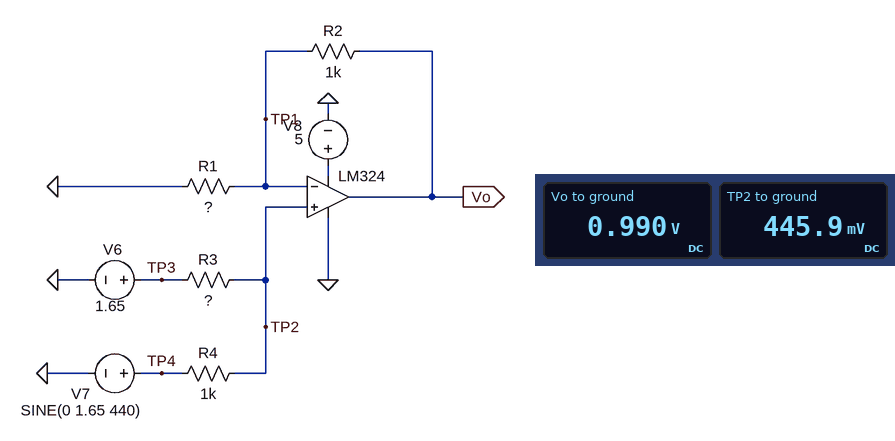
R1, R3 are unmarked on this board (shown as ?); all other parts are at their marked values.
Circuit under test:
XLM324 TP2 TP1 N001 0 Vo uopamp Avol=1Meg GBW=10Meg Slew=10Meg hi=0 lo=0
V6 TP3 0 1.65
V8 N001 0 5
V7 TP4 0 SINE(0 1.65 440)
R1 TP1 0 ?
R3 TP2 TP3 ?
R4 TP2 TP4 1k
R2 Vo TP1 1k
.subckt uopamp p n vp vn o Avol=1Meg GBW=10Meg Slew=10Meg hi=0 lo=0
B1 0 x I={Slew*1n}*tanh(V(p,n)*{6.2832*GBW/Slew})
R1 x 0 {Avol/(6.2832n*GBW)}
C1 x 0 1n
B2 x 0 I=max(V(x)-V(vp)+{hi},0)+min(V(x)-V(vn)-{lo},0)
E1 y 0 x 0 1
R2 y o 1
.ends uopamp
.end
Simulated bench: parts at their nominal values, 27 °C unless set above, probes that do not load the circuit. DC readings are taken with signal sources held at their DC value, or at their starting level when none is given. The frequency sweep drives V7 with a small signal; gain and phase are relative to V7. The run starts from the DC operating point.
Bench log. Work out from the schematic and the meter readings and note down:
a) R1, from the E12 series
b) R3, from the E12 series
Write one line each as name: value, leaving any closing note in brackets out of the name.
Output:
R1, from the E12 series: 820 Ω
R3, from the E12 series: 2.7 kΩ
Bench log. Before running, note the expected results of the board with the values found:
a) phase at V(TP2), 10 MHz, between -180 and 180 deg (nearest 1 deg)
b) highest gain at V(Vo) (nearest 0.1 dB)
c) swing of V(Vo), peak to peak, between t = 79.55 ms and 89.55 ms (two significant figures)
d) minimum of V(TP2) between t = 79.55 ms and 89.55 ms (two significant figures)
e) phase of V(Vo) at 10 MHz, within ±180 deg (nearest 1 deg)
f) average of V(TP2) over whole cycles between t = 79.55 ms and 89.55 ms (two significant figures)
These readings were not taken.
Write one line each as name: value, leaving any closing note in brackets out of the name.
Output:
phase at V(TP2), 10 MHz, between -180 and 180 deg: 0 deg
highest gain at V(Vo): 4.2 dB
swing of V(Vo), peak to peak, between t = 79.55 ms and 89.55 ms: 3.7 V
minimum of V(TP2) between t = 79.55 ms and 89.55 ms: -760 mV
phase of V(Vo) at 10 MHz, within ±180 deg: -66 deg
average of V(TP2) over whole cycles between t = 79.55 ms and 89.55 ms: 450 mV
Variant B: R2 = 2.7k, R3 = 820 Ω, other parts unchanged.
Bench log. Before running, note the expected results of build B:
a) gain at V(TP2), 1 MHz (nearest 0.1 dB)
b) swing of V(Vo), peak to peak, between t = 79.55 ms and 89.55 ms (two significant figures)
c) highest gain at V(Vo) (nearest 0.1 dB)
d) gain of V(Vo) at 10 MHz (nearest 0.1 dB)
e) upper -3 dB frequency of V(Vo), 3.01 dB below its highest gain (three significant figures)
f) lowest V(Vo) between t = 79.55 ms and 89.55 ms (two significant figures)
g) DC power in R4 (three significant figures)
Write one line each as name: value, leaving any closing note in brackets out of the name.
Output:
gain at V(TP2), 1 MHz: -6.9 dB
swing of V(Vo), peak to peak, between t = 79.55 ms and 89.55 ms: 4.3 V
highest gain at V(Vo): 5.7 dB
gain of V(Vo) at 10 MHz: -7.2 dB
upper -3 dB frequency of V(Vo), 3.01 dB below its highest gain: 2.33 MHz
lowest V(Vo) between t = 79.55 ms and 89.55 ms: 700 mV
DC power in R4: 822 µW
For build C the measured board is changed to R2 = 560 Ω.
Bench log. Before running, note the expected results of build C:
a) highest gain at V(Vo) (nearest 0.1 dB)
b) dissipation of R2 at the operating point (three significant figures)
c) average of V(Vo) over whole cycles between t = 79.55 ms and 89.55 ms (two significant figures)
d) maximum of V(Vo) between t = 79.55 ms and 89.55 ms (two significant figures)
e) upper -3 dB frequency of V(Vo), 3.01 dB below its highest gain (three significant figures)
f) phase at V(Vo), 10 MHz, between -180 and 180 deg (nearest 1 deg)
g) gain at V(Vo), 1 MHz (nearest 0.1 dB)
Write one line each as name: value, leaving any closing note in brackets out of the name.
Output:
highest gain at V(Vo): 1.8 dB
dissipation of R2 at the operating point: 166 µW
average of V(Vo) over whole cycles between t = 79.55 ms and 89.55 ms: 1.1 V
maximum of V(Vo) between t = 79.55 ms and 89.55 ms: 2.8 V
upper -3 dB frequency of V(Vo), 3.01 dB below its highest gain: 5.94 MHz
phase at V(Vo), 10 MHz, between -180 and 180 deg: -59 deg
gain at V(Vo), 1 MHz: 1.7 dB
